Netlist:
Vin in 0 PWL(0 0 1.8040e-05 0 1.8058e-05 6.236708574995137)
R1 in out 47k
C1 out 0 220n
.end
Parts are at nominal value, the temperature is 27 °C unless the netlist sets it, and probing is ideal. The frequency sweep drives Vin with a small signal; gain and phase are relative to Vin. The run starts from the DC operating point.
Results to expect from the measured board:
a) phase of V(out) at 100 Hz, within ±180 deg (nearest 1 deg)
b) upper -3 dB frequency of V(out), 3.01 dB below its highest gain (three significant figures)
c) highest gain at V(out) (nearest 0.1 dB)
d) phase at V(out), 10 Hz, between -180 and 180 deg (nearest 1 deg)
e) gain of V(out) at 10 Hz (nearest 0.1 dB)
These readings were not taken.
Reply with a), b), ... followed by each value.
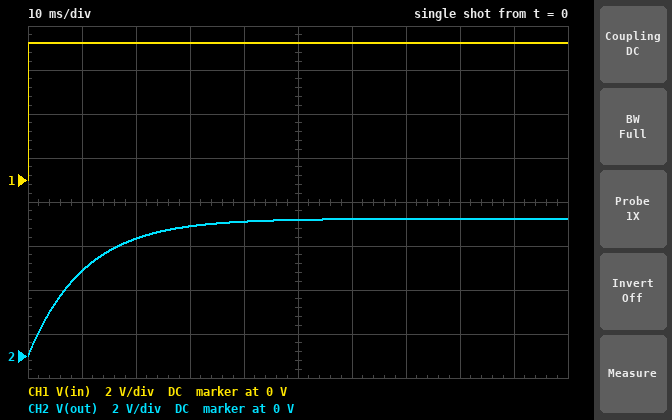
a) -81 deg
b) 15.4 Hz
c) 0 dB
d) -33 deg
e) -1.5 dB
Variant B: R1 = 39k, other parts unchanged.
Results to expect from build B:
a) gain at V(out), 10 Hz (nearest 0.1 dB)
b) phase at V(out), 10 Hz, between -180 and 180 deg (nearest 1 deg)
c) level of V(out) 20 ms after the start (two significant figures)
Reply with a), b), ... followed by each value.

a) -1.1 dB
b) -28 deg
c) 5.6 V
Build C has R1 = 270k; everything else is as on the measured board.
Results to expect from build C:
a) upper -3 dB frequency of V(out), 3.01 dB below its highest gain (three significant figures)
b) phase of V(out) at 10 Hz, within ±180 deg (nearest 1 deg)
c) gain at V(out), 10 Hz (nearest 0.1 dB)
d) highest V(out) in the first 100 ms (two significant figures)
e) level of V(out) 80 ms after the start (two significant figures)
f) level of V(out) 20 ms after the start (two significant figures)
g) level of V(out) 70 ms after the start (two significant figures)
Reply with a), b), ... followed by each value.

a) 2.68 Hz
b) -75 deg
c) -11.7 dB
d) 5.1 V
e) 4.6 V
f) 1.8 V
g) 4.3 V
